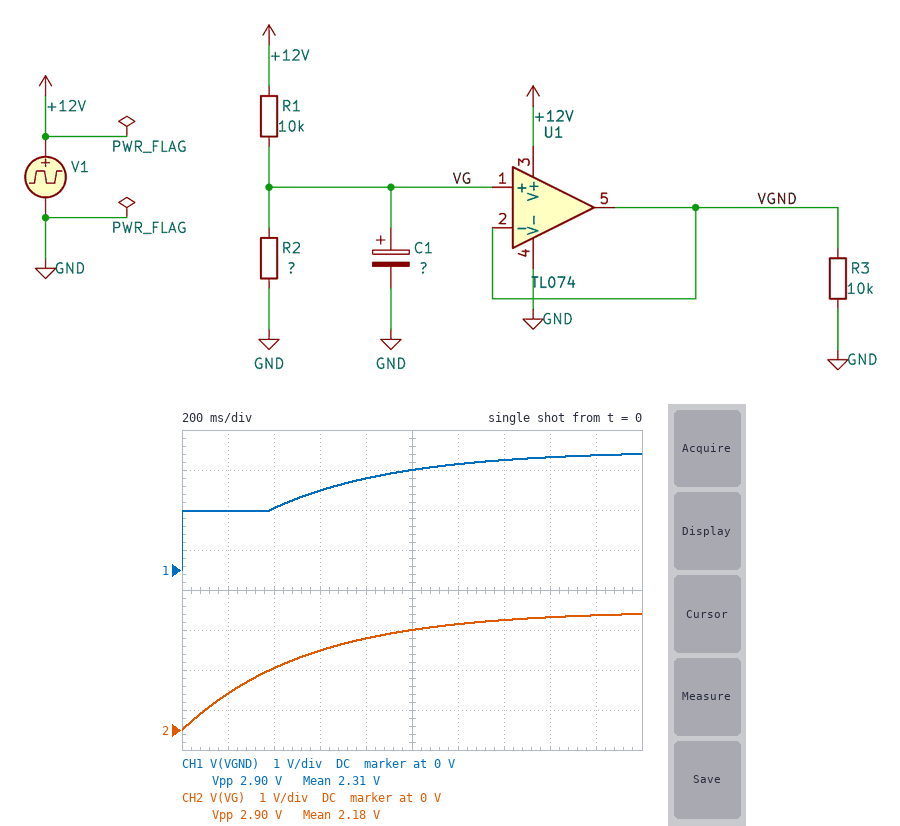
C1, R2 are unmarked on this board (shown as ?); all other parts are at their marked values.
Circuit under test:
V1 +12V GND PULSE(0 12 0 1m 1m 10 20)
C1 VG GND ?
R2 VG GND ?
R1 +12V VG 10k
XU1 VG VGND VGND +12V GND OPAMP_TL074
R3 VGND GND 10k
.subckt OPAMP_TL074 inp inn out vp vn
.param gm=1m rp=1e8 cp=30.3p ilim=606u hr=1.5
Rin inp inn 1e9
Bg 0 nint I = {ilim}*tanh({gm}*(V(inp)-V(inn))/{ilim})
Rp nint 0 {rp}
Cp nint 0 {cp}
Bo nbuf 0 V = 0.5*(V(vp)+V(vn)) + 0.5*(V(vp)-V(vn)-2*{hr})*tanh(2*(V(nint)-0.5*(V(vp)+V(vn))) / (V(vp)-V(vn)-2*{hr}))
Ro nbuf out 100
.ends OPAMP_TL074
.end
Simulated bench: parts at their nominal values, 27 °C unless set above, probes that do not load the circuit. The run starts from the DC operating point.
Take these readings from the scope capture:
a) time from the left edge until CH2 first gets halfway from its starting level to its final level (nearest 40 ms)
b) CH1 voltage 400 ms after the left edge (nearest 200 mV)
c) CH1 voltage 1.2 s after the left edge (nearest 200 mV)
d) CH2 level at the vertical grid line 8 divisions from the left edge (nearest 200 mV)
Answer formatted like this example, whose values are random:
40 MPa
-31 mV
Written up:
360 ms
1.6 V
2.6 V
2.8 V
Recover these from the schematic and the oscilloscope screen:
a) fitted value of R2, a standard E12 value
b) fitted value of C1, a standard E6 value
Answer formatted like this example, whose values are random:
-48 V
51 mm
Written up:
3.3 kΩ
220 µF
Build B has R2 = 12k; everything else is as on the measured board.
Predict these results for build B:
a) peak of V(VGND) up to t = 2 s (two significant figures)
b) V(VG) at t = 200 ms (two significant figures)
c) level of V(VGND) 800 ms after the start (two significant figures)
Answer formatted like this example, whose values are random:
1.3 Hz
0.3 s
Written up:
5.3 V
1.0 V
3.2 V
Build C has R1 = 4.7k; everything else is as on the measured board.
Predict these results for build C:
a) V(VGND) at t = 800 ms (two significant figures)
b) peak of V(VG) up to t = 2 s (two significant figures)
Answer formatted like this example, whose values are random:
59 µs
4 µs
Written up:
4.2 V
4.9 V
